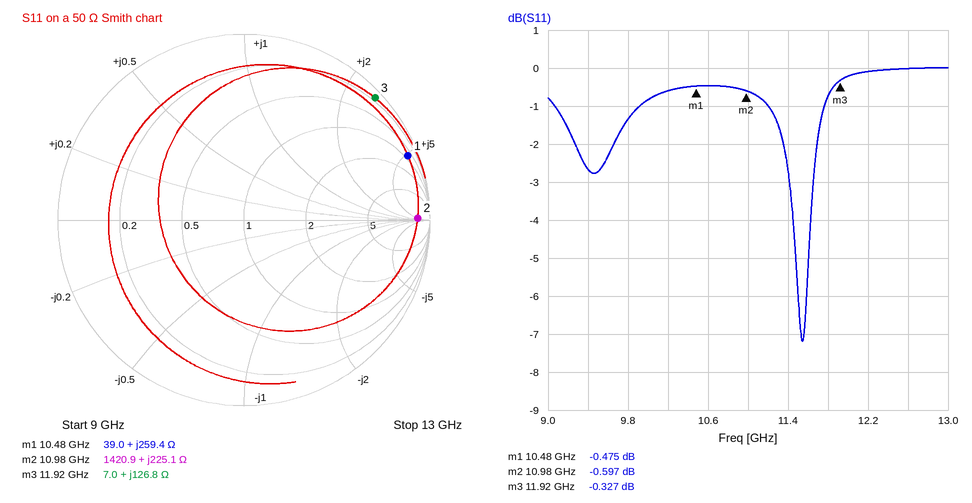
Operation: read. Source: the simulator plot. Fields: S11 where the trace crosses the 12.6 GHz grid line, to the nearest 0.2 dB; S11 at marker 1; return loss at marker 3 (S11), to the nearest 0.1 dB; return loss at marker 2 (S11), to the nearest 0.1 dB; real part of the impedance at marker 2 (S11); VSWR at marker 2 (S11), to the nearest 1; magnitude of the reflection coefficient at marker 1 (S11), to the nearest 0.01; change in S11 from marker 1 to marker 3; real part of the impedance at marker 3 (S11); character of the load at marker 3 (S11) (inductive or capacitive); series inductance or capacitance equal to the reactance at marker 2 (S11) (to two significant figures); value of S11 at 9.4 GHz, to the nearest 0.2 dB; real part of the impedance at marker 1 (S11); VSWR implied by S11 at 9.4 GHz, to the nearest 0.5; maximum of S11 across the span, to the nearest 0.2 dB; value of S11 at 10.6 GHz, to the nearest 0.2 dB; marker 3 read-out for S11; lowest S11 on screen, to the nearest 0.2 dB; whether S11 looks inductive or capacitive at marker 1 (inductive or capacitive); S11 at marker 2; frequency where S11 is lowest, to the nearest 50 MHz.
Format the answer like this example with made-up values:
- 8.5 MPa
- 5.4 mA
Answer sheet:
- 0.0 dB
- -0.475 dB
- 0.3 dB
- 0.6 dB
- 1420.9 Ω
- 29
- 0.95
- 0.148 dB
- 7.0 Ω
- inductive
- 3.3 nH
- -2.6 dB
- 39.0 Ω
- 6.5
- 0.0 dB
- -0.4 dB
- -0.327 dB
- -7.2 dB
- inductive
- -0.597 dB
- 11.55 GHz
